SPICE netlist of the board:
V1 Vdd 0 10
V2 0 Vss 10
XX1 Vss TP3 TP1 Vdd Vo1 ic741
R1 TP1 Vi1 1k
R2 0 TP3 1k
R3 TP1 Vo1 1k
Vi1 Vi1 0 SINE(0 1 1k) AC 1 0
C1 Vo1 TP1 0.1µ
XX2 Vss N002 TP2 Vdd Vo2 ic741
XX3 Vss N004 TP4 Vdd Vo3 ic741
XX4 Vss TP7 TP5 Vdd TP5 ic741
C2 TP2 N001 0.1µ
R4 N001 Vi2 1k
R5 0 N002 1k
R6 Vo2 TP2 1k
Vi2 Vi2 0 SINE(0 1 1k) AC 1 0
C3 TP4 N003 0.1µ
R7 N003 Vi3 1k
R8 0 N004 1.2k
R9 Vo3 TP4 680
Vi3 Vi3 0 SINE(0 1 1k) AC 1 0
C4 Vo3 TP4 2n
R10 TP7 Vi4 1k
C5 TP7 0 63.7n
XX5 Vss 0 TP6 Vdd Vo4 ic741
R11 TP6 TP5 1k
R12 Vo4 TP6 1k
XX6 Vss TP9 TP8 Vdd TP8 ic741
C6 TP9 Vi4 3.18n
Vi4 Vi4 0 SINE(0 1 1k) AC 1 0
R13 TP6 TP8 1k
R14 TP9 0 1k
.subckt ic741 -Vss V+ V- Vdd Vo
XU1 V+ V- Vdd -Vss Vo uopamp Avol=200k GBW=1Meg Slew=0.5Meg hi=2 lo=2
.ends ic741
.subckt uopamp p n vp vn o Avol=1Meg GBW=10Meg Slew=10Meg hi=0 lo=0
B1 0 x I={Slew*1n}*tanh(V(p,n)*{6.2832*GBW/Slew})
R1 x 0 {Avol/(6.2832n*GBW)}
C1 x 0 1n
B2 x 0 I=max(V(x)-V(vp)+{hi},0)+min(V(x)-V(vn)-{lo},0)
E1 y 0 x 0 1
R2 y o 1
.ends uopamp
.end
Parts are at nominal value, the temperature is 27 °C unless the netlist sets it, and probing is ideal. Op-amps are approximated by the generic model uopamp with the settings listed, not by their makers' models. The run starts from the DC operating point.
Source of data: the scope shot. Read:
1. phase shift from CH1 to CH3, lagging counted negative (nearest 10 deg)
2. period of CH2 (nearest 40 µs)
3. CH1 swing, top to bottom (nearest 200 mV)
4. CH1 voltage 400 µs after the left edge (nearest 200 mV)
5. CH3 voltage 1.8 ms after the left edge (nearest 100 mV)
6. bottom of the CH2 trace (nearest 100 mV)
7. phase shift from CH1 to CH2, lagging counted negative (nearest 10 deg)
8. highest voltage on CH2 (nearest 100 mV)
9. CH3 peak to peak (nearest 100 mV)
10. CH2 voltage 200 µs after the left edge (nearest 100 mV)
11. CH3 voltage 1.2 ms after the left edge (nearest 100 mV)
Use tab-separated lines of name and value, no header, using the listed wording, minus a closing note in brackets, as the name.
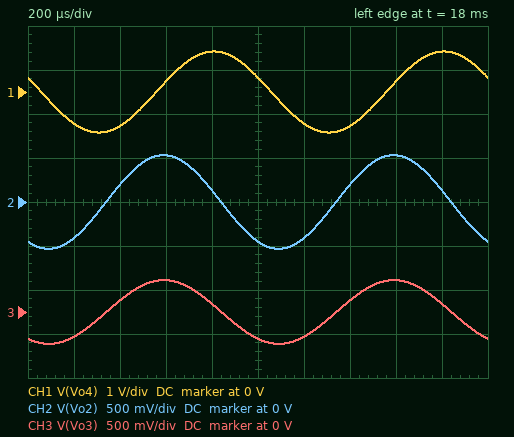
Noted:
phase shift from CH1 to CH3, lagging counted negative	80 deg
period of CH2	1.00 ms
CH1 swing, top to bottom	1.8 V
CH1 voltage 400 µs after the left edge	-800 mV
CH3 voltage 1.8 ms after the left edge	100 mV
bottom of the CH2 trace	-500 mV
phase shift from CH1 to CH2, lagging counted negative	80 deg
highest voltage on CH2	500 mV
CH3 peak to peak	700 mV
CH2 voltage 200 µs after the left edge	-400 mV
CH3 voltage 1.2 ms after the left edge	-300 mV
